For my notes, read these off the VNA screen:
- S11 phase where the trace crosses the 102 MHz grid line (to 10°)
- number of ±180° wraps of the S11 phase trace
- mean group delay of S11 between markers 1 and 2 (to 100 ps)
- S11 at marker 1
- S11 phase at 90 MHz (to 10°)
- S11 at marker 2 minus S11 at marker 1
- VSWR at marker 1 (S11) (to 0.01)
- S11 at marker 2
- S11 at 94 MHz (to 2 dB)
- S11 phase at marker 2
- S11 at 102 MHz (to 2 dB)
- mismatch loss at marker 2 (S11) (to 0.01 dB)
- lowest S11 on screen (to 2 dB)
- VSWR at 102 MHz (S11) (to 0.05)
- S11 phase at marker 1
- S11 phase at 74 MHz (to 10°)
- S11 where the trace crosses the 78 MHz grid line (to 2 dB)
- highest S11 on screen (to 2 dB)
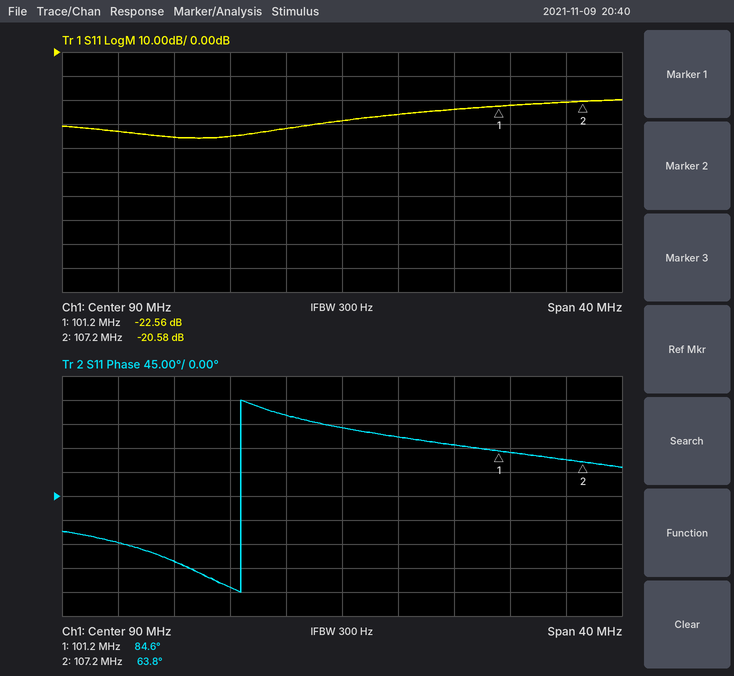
80°
1
9.6 ns
-22.56 dB
130°
1.98 dB
1.16
-20.58 dB
-26 dB
63.8°
-22 dB
0.04 dB
-36 dB
1.15
84.6°
-90°
-36 dB
-20 dB
